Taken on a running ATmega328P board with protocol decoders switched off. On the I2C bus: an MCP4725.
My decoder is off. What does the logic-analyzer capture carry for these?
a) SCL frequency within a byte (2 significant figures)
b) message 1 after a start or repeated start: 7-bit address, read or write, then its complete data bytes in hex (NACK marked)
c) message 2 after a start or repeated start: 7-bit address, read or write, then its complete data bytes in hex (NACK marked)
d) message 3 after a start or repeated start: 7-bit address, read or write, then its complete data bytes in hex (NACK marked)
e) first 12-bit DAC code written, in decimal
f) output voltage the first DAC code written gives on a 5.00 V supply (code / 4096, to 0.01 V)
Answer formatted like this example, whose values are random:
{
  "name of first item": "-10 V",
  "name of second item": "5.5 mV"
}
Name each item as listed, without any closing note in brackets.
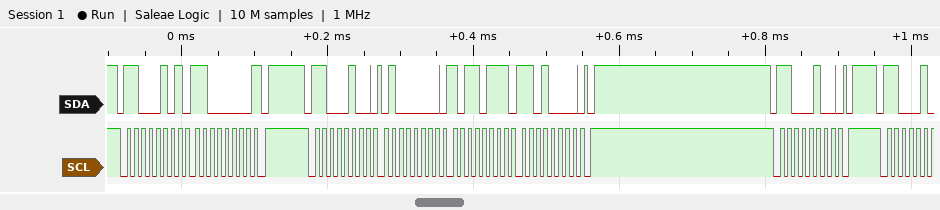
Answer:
{
  "SCL frequency within a byte": "100 kHz",
  "message 1 after a start or repeated start: 7-bit address, read or write, then its complete data bytes in hex": "0x62 read: C0 NACK",
  "message 2 after a start or repeated start: 7-bit address, read or write, then its complete data bytes in hex": "0x62 write: 40 B7 D0",
  "message 3 after a start or repeated start: 7-bit address, read or write, then its complete data bytes in hex": "0x62 write",
  "first 12-bit DAC code written, in decimal": "2941",
  "output voltage the first DAC code written gives on a 5.00 V supply": "3.59 V"
}
